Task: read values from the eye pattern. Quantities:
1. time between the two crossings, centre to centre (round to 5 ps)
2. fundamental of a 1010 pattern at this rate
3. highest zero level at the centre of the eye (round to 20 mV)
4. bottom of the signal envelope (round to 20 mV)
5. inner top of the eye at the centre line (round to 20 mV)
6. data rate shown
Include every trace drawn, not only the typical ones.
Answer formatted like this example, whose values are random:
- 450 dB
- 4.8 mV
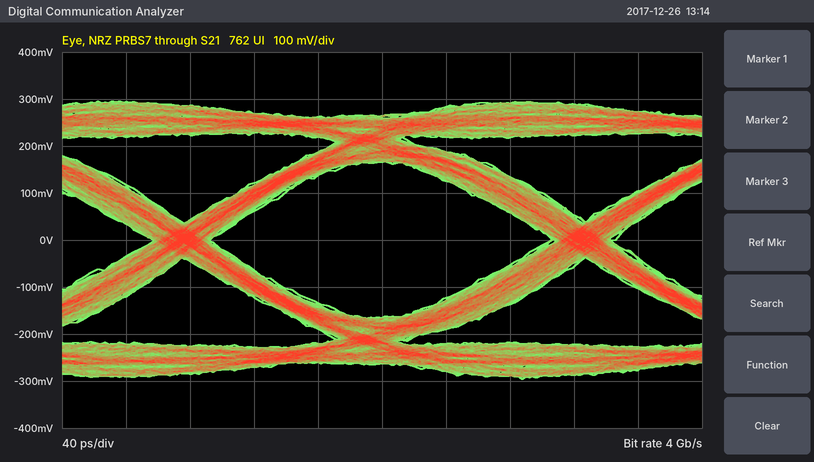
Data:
- 250 ps
- 2 GHz
- -160 mV
- -300 mV
- 160 mV
- 4 Gb/s
